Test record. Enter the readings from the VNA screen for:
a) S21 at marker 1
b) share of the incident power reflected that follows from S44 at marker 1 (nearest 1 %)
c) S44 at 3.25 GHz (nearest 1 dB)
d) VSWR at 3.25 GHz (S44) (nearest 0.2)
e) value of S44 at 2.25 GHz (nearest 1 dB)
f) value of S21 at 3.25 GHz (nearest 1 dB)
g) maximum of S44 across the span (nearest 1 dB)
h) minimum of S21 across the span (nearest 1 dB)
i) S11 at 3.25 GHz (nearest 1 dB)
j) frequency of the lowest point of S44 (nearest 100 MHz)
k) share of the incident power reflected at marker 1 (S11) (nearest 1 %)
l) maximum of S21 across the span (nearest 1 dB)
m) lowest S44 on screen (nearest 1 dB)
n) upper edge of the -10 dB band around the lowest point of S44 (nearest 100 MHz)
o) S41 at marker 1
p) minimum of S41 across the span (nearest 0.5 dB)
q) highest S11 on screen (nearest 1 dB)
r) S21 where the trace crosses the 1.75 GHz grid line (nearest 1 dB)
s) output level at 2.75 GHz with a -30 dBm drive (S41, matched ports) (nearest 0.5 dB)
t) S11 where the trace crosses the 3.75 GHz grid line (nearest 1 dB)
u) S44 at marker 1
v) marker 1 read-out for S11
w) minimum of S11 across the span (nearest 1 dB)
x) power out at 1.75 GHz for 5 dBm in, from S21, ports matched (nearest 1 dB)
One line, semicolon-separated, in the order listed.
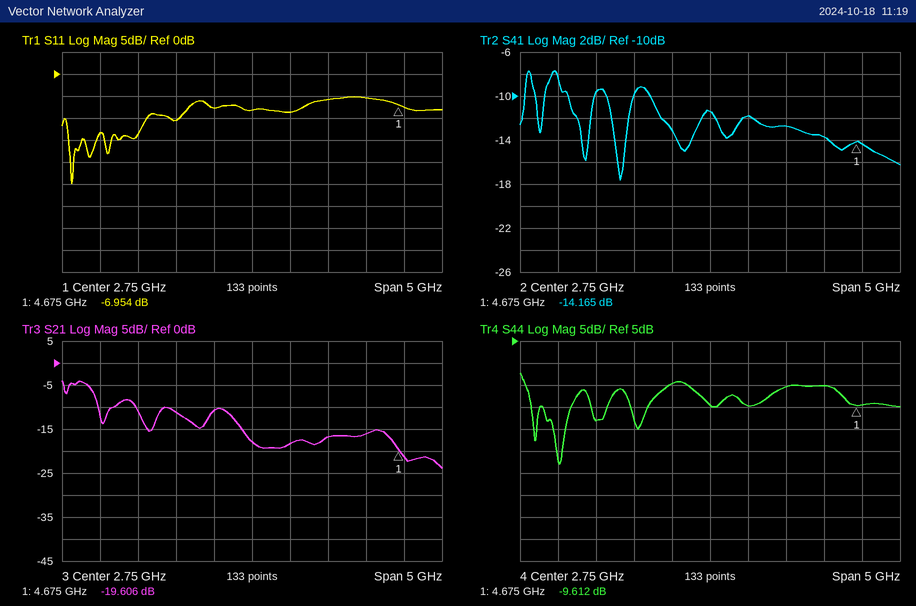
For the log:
-19.606 dB; 11 %; -10 dB; 2.0; -5 dB; -18 dB; -2 dB; -24 dB; -9 dB; 800 MHz; 20 %; -4 dB; -23 dB; 900 MHz; -14.165 dB; -17.5 dB; -5 dB; -11 dB; -41.5 dBm; -6 dB; -9.612 dB; -6.954 dB; -25 dB; -6 dBm
